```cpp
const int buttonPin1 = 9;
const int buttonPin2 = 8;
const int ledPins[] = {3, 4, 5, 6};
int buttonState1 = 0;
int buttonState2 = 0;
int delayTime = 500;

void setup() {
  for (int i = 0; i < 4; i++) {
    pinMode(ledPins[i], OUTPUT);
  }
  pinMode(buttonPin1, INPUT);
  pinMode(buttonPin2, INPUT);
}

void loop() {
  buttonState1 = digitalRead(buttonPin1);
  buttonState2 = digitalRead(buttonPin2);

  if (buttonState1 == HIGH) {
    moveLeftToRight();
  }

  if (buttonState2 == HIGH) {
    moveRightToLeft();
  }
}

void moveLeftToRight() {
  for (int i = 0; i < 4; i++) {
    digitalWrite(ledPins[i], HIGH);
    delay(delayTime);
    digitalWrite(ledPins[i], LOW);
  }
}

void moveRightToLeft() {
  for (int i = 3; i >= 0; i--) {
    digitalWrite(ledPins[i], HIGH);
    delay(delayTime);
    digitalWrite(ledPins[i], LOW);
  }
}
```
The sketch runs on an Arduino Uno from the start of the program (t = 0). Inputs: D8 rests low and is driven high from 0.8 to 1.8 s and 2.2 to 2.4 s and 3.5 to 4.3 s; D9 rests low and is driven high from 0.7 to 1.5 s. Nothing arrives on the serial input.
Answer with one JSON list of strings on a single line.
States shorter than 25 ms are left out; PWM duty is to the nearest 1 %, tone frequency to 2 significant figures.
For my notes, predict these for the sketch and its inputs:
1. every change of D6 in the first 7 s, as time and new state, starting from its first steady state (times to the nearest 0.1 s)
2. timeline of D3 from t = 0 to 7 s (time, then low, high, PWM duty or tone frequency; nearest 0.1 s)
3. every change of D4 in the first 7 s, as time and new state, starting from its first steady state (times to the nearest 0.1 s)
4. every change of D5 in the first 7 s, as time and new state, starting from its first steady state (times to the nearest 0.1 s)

["0 s low; 2.2 s high; 2.7 s low; 3.5 s high; 4 s low", "0 s low; 0.7 s high; 1.2 s low; 5 s high; 5.5 s low", "0 s low; 1.2 s high; 1.7 s low; 4.5 s high; 5 s low", "0 s low; 1.7 s high; 2.2 s low; 4 s high; 4.5 s low"]
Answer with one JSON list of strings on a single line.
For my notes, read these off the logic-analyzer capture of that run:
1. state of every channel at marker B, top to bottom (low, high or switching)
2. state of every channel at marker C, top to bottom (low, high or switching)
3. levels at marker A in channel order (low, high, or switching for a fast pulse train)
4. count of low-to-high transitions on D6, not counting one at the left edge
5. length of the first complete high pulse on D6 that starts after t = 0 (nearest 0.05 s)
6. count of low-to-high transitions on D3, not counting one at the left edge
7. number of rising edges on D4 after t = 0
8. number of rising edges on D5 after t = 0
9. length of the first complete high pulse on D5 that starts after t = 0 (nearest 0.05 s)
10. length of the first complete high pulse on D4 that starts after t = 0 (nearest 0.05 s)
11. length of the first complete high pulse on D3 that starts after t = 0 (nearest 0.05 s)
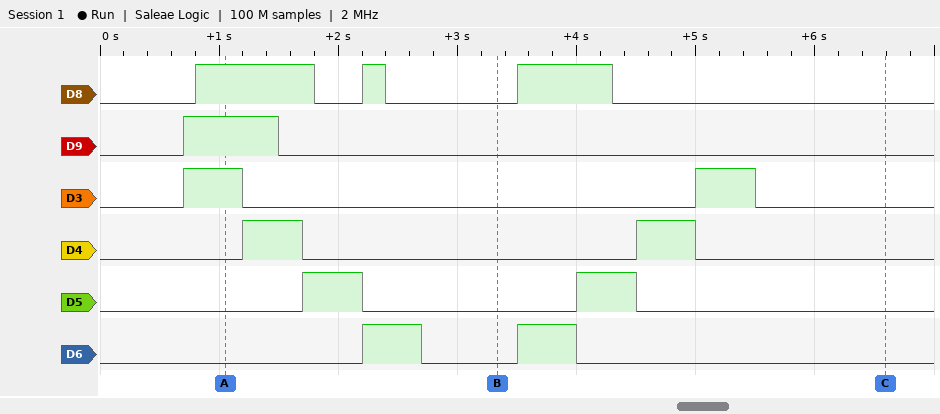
["D8 low, D9 low, D3 low, D4 low, D5 low, D6 low", "D8 low, D9 low, D3 low, D4 low, D5 low, D6 low", "D8 high, D9 high, D3 high, D4 low, D5 low, D6 low", "2", "0.50 s", "2", "2", "2", "0.50 s", "0.50 s", "0.50 s"]
